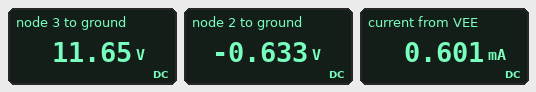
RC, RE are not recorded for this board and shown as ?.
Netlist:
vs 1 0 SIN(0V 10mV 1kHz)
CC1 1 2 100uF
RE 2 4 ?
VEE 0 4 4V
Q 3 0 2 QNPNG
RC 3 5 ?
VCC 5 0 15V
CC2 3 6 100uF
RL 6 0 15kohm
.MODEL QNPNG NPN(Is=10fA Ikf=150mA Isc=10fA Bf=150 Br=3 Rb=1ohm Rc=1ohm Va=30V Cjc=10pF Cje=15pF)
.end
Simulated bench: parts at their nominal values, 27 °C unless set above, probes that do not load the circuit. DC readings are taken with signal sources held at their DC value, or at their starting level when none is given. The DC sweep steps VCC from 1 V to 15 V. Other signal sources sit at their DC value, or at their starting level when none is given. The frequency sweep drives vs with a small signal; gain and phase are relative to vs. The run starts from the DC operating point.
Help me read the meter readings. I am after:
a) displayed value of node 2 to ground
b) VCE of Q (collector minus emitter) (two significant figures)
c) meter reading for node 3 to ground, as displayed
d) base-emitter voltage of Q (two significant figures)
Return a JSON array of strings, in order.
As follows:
["-0.633 V", "12 V", "11.65 V", "630 mV"]
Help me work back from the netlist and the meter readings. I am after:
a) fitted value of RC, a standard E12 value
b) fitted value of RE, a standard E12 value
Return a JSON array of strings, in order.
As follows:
["5.6 kΩ", "5.6 kΩ"]
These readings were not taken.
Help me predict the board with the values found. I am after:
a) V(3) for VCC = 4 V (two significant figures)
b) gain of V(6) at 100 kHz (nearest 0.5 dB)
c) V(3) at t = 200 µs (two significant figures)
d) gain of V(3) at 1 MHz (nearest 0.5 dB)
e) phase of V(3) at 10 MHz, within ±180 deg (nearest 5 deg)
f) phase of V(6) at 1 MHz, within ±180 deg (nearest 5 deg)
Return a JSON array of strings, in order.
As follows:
["660 mV", "39.0 dB", "12 V", "39.0 dB", "-45 deg", "-5 deg"]
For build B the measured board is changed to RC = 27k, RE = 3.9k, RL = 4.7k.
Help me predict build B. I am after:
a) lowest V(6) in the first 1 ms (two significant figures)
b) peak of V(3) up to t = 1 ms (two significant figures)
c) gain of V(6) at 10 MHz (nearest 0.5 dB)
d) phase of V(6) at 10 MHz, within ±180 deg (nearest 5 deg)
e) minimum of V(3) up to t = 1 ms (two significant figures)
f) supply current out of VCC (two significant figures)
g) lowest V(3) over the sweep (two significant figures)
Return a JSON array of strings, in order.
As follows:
["-14 mV", "-630 mV", "3.5 dB", "0 deg", "-660 mV", "580 µA", "-680 mV"]
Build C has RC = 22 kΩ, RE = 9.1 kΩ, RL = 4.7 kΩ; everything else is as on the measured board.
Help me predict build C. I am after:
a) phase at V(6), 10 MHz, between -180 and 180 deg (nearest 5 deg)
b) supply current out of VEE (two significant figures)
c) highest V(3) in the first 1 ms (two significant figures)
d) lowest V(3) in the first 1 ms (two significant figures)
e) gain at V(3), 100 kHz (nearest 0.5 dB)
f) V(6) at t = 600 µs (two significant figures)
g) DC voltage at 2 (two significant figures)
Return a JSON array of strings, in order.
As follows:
["-50 deg", "370 µA", "7.3 V", "6.2 V", "34.5 dB", "-370 mV", "-620 mV"]
